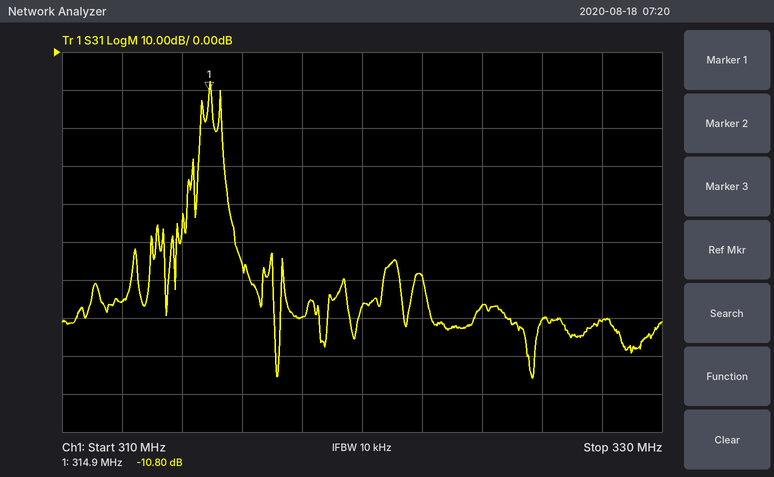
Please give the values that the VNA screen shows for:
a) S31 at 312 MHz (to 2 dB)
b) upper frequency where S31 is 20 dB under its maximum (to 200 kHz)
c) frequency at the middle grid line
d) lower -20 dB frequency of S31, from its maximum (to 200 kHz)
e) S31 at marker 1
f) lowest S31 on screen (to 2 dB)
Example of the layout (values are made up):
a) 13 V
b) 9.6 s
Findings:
a) -66 dB
b) 315.4 MHz
c) 320 MHz
d) 314.6 MHz
e) -10.80 dB
f) -86 dB
